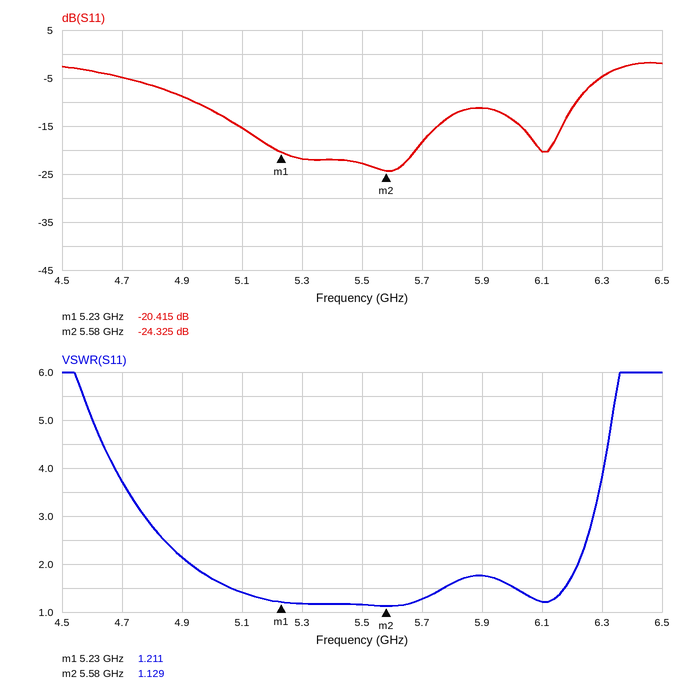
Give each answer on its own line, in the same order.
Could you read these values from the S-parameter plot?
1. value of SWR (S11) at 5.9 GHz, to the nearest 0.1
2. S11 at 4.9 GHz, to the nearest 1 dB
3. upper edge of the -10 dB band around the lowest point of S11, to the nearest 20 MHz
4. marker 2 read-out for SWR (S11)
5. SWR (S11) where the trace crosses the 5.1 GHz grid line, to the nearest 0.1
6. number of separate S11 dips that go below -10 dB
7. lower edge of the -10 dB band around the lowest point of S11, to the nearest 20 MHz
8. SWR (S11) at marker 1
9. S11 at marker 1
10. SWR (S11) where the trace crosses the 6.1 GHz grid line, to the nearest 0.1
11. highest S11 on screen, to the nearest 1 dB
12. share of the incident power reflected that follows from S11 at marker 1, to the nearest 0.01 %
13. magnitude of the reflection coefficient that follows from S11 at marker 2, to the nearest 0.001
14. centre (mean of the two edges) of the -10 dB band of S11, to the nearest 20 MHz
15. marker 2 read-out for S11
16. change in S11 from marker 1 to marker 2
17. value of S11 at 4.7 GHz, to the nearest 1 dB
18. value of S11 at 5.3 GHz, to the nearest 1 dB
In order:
1.8
-9 dB
6.22 GHz
1.129
1.4
2
4.94 GHz
1.211
-20.415 dB
1.2
-2 dB
0.91 %
0.061
5.58 GHz
-24.325 dB
-3.910 dB
-5 dB
-22 dB
